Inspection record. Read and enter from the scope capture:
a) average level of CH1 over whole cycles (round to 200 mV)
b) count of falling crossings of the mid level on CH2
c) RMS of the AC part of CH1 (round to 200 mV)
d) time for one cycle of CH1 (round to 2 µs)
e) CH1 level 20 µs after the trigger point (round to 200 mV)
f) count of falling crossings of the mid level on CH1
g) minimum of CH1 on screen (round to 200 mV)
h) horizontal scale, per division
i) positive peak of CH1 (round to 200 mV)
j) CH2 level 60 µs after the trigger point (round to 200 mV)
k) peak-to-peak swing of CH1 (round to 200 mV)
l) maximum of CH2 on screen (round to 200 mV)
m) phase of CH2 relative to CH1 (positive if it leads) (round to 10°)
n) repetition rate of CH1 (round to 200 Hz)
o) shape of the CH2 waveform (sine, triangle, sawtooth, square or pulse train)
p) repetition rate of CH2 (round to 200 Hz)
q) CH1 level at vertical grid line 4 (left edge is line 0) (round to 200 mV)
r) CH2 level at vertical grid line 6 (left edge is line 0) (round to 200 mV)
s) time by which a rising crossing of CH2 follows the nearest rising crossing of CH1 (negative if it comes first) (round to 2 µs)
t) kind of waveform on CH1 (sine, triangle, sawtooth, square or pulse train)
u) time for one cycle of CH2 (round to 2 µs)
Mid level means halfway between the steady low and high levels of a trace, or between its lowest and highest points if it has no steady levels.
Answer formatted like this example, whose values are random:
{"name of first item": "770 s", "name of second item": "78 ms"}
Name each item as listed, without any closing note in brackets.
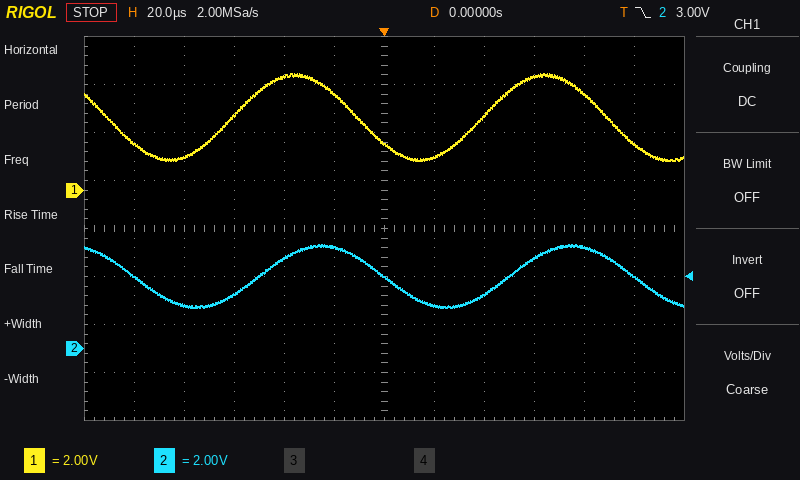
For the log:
{"average level of CH1 over whole cycles": "3.0 V", "count of falling crossings of the mid level on CH2": "3", "RMS of the AC part of CH1": "1.2 V", "time for one cycle of CH1": "100 µs", "CH1 level 20 µs after the trigger point": "1.4 V", "count of falling crossings of the mid level on CH1": "3", "minimum of CH1 on screen": "1.2 V", "horizontal scale, per division": "20 µs", "positive peak of CH1": "4.8 V", "CH2 level 60 µs after the trigger point": "3.8 V", "peak-to-peak swing of CH1": "3.6 V", "maximum of CH2 on screen": "4.4 V", "phase of CH2 relative to CH1 (positive if it leads)": "-40°", "repetition rate of CH1": "10.0 kHz", "shape of the CH2 waveform": "sine", "repetition rate of CH2": "10.0 kHz", "CH1 level at vertical grid line 4 (left edge is line 0)": "4.8 V", "CH2 level at vertical grid line 6 (left edge is line 0)": "3.0 V", "time by which a rising crossing of CH2 follows the nearest rising crossing of CH1 (negative if it comes first)": "+10 µs", "kind of waveform on CH1": "sine", "time for one cycle of CH2": "100 µs"}
